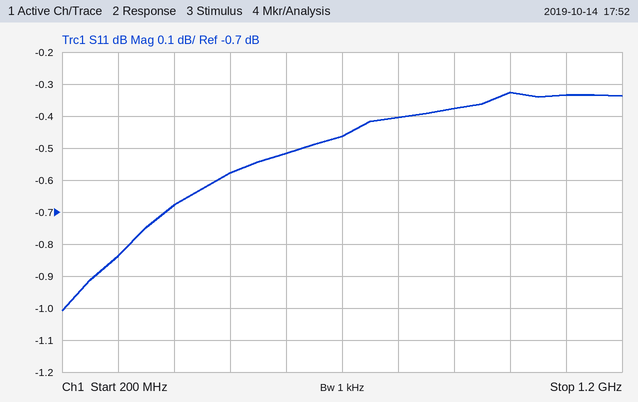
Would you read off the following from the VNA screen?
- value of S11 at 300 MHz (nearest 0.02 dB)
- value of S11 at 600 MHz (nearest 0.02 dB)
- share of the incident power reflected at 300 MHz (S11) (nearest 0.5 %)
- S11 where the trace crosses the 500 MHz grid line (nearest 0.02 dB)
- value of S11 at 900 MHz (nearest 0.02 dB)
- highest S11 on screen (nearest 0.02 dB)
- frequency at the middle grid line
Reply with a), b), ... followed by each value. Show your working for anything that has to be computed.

a) -0.84 dB
b) -0.52 dB
c) 10^(-0.84/10) ≈ 82.4 %, so 82.5 % to the nearest 0.5 %
d) -0.58 dB
e) -0.38 dB
f) -0.32 dB
g) 700 MHz
